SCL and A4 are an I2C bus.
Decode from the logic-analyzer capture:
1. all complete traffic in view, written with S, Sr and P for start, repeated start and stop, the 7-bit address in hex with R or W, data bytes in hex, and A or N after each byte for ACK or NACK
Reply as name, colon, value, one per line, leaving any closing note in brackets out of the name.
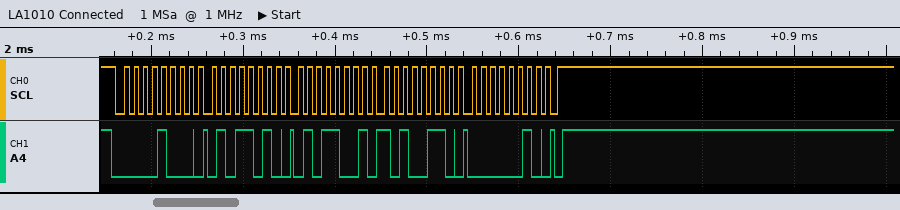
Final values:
all complete traffic in view, written with S, Sr and P for start, repeated start and stop, the 7-bit address in hex with R or W, data bytes in hex, and A or N after each byte for ACK or NACK: S 04W A 5A A 59 A A6 A 02 A P
